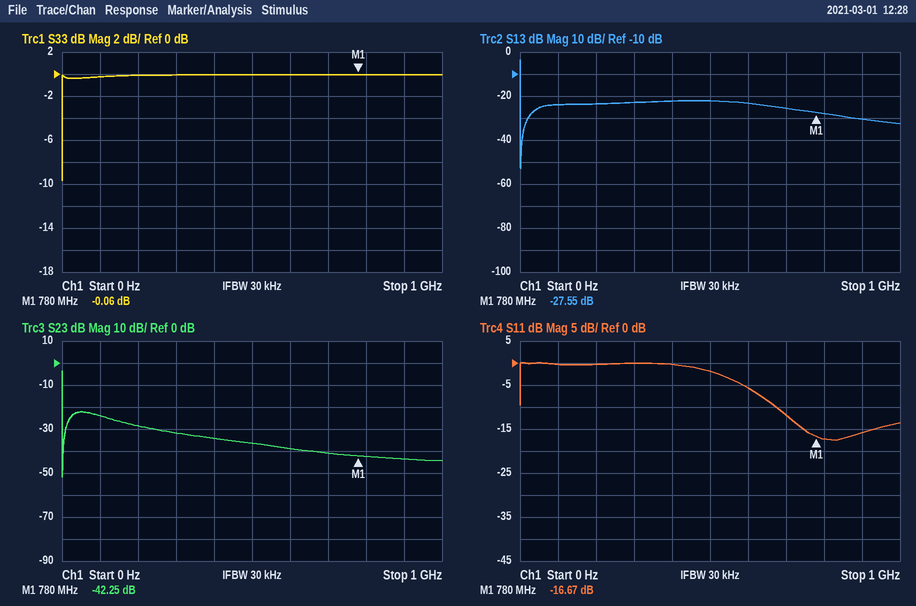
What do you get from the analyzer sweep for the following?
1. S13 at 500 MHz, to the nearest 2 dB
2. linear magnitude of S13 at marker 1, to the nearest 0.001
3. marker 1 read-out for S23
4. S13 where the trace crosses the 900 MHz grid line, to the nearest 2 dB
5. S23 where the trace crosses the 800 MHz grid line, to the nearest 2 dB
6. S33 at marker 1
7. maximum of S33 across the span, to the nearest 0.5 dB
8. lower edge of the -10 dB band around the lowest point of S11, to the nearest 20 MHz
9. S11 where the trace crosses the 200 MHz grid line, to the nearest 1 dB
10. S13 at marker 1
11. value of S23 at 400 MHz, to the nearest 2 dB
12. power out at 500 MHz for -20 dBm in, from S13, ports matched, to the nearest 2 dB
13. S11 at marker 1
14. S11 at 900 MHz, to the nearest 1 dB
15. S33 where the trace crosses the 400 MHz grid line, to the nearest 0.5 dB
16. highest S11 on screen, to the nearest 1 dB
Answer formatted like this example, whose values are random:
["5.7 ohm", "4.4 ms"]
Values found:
["-22 dB", "0.042", "-42.25 dB", "-30 dB", "-42 dB", "-0.06 dB", "0.0 dB", "680 MHz", "0 dB", "-27.55 dB", "-34 dB", "-42 dBm", "-16.67 dB", "-16 dB", "0.0 dB", "0 dB"]
